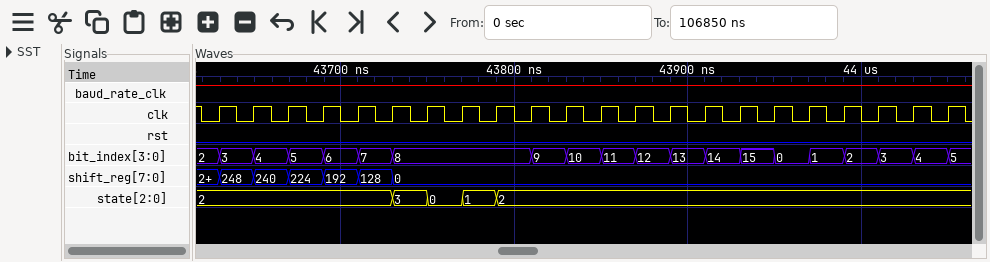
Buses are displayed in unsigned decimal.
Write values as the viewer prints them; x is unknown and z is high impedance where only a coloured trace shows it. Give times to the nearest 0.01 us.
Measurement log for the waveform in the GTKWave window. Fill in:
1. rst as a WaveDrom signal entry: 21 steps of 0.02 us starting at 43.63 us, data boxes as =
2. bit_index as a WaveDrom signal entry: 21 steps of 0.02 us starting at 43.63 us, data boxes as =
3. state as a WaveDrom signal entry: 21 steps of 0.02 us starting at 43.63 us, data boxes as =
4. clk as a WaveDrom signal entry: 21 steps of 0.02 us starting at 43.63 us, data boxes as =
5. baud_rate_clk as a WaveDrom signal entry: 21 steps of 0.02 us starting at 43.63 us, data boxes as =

{name: 'rst', wave: '0....................'}
{name: 'bit_index', wave: '======...============', data: '3 4 5 6 7 8 9 10 11 12 13 14 15 0 1 2 3 4'}
{name: 'state', wave: '=....====............', data: '2 3 0 1 2'}
{name: 'clk', wave: 'p....................'}
{name: 'baud_rate_clk', wave: '1....................'}
